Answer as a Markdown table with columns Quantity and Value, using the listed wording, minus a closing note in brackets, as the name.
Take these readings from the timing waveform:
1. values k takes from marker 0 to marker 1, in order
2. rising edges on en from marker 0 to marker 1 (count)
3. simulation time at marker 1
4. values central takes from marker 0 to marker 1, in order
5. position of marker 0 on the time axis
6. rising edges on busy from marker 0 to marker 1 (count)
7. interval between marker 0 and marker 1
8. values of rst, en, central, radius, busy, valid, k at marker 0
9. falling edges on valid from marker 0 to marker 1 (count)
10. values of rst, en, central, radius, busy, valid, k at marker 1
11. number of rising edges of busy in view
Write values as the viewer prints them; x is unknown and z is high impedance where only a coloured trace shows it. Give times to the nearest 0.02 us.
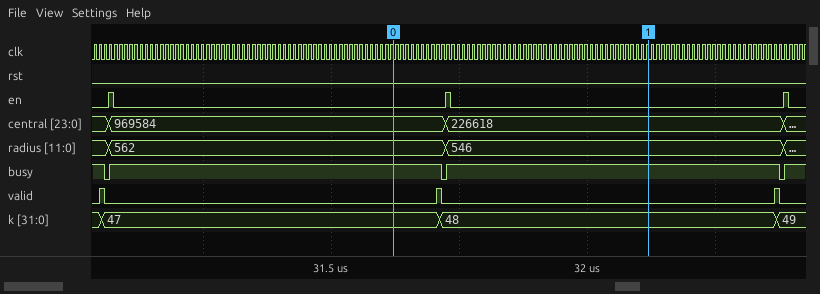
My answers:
| Quantity | Value |
|---|---|
| values k takes from marker 0 to marker 1, in order | 47, 48 |
| rising edges on en from marker 0 to marker 1 | 1 |
| simulation time at marker 1 | 32.12 us |
| values central takes from marker 0 to marker 1, in order | 969584, 226618 |
| position of marker 0 on the time axis | 31.62 us |
| rising edges on busy from marker 0 to marker 1 | 1 |
| interval between marker 0 and marker 1 | 0.5 us |
| values of rst, en, central, radius, busy, valid, k at marker 0 | rst=0, en=0, central=969584, radius=562, busy=1, valid=0, k=47 |
| falling edges on valid from marker 0 to marker 1 | 1 |
| values of rst, en, central, radius, busy, valid, k at marker 1 | rst=0, en=0, central=226618, radius=546, busy=1, valid=0, k=48 |
| number of rising edges of busy in view | 3 |
